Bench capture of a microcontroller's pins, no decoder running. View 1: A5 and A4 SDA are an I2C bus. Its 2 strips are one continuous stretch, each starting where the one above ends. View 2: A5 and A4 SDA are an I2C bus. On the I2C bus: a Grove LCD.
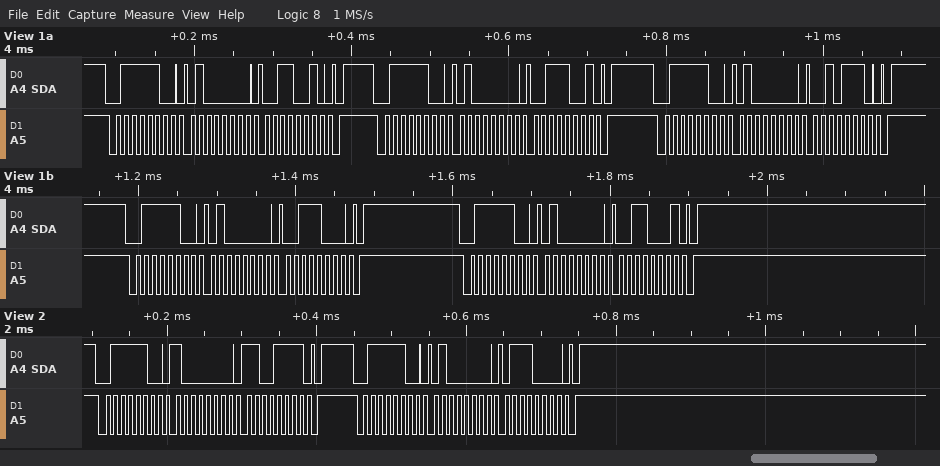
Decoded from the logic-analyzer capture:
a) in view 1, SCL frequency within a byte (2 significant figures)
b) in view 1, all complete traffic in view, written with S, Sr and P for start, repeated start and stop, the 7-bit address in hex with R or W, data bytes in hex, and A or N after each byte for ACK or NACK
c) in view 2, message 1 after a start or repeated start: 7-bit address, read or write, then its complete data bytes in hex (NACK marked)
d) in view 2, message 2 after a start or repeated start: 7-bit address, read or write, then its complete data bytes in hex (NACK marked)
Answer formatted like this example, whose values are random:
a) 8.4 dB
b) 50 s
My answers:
a) 100 kHz
b) S 3EW A 40 A 32 A P S 3EW A 40 A 39 A P S 3EW A 40 A 2E A P S 3EW A 40 A 38 A P S 3EW A 40 A 31 A P
c) 0x3E write: 80 CF
d) 0x3E write: 40 70
